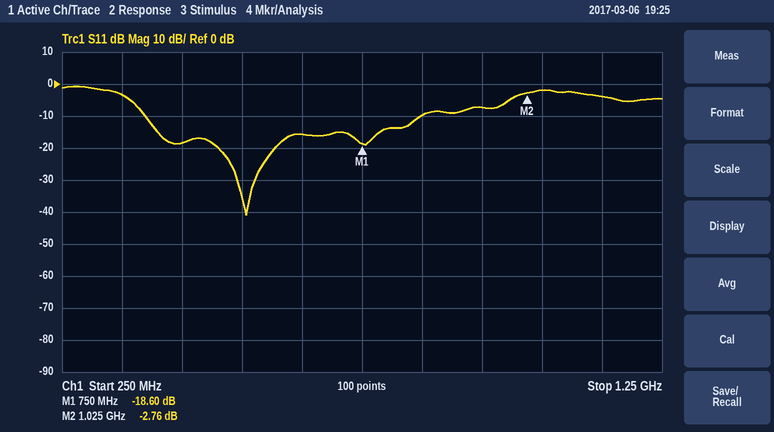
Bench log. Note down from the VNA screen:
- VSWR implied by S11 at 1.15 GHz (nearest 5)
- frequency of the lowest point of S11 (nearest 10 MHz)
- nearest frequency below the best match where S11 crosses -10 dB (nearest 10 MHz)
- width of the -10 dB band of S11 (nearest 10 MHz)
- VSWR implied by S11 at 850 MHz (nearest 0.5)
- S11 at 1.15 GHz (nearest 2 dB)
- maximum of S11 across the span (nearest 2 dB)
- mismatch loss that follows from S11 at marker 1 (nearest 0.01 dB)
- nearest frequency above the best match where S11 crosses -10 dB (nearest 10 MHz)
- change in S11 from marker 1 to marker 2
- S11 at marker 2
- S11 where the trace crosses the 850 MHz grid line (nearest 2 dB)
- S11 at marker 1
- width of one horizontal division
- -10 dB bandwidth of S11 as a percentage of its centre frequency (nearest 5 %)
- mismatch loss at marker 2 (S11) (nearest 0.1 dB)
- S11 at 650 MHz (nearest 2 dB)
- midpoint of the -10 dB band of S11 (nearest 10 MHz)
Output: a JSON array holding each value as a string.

["5", "560 MHz", "390 MHz", "460 MHz", "2.0", "-4 dB", "0 dB", "0.06 dB", "850 MHz", "15.84 dB", "-2.76 dB", "-10 dB", "-18.60 dB", "100 MHz", "75 %", "3.3 dB", "-16 dB", "620 MHz"]
